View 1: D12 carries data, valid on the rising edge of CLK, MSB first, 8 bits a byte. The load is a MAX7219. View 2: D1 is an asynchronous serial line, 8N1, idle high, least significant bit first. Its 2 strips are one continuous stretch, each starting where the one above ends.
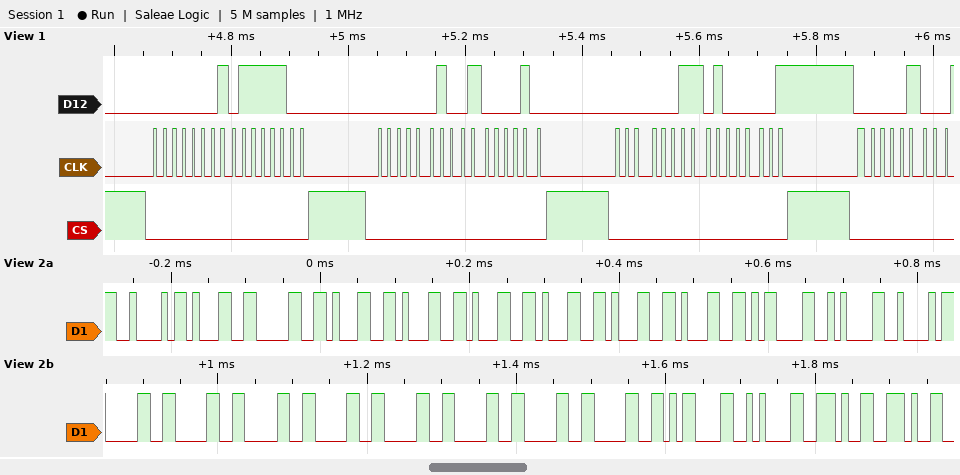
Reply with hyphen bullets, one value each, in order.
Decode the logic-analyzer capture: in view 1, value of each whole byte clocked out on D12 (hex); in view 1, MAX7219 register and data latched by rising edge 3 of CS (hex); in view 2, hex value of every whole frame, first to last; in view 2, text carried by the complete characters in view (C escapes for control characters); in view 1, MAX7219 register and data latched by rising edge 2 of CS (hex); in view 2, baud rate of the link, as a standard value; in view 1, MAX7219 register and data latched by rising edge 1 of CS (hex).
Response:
- 0x01 0x7C 0x02 0x42 0x03 0x41 0x04
- register 0x3, data 0x41
- 42 31 30 31 31 31 31 31 31 0D 0A 42 30 30 30 30 30 30 30 30 0D 0A 2E 2E
- "B10111111\r\nB00000000\r\n.."
- register 0x2, data 0x42
- 115200 baud
- register 0x1, data 0x7C
